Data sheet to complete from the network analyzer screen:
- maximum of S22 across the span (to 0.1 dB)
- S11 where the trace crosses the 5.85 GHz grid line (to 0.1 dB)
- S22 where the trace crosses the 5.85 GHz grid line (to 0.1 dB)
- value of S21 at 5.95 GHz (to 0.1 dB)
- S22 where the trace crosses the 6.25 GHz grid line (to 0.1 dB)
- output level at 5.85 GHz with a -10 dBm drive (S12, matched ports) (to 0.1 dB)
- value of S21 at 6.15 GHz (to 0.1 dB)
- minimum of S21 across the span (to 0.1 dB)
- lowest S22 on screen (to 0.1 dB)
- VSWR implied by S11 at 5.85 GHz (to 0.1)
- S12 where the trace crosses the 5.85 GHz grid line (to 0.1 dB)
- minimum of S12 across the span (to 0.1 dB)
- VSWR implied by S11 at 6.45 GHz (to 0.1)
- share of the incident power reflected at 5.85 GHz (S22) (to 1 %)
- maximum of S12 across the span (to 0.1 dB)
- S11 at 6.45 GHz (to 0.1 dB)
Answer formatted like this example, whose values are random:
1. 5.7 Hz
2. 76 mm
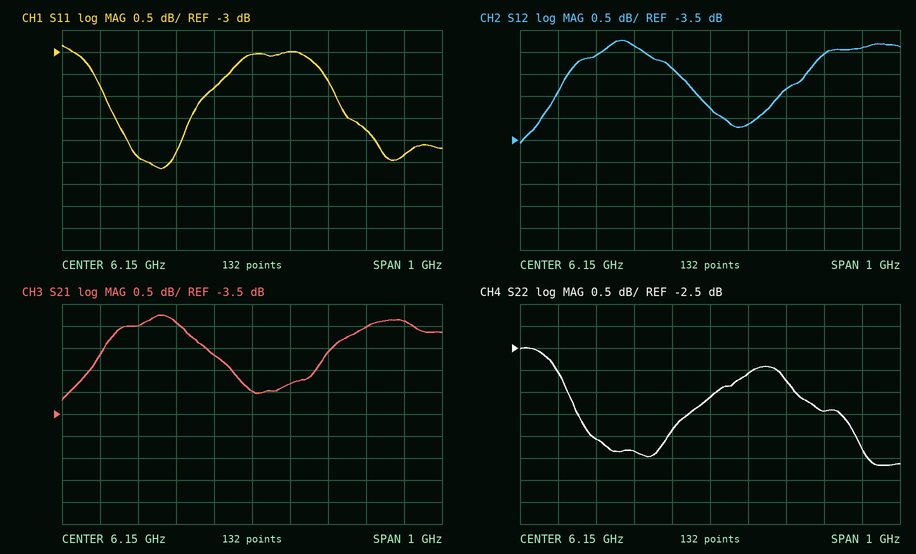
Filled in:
1. -2.5 dB
2. -5.4 dB
3. -4.6 dB
4. -1.4 dB
5. -3.1 dB
6. -11.6 dBm
7. -3.0 dB
8. -3.2 dB
9. -5.2 dB
10. 3.3
11. -1.6 dB
12. -3.6 dB
13. 3.7
14. 35 %
15. -1.2 dB
16. -4.8 dB
